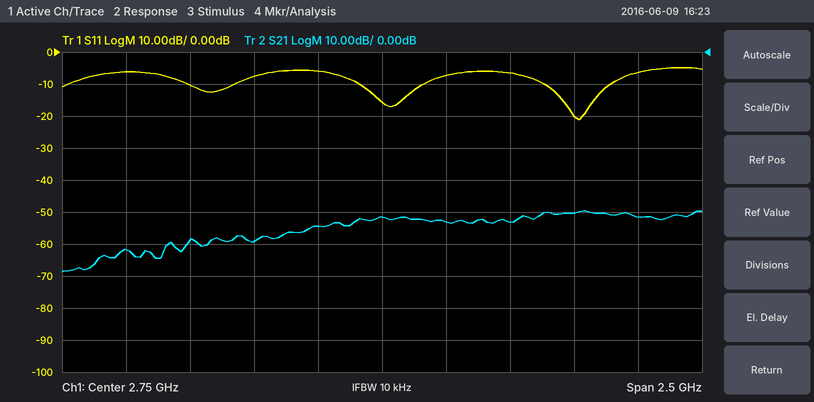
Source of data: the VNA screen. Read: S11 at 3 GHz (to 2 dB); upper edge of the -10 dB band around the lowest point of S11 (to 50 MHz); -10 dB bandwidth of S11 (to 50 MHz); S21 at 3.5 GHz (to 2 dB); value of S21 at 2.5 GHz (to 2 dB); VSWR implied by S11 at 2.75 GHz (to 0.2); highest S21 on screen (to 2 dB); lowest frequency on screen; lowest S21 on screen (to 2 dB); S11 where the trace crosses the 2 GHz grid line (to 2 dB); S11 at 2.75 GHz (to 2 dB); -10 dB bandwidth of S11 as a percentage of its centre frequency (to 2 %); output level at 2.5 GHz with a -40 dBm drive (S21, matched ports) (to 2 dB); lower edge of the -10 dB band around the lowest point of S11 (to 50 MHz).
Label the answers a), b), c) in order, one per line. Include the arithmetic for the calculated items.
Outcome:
a) -8 dB
b) 3.65 GHz
c) 3.65 GHz − 3.40 GHz = 250 MHz
d) -50 dB
e) -54 dB
f) |Γ| = 10^(-16/20) = 0.1585; VSWR = (1 + 0.1585)/(1 − 0.1585) ≈ 1.4
g) -50 dB
h) 1.5 GHz
i) -68 dB
j) -10 dB
k) -16 dB
l) 250 MHz / 3.525 GHz ≈ 7.09 %, so 8 % to the nearest 2 %
m) -40 dBm + (-54 dB) = -94 dBm
n) 3.40 GHz
